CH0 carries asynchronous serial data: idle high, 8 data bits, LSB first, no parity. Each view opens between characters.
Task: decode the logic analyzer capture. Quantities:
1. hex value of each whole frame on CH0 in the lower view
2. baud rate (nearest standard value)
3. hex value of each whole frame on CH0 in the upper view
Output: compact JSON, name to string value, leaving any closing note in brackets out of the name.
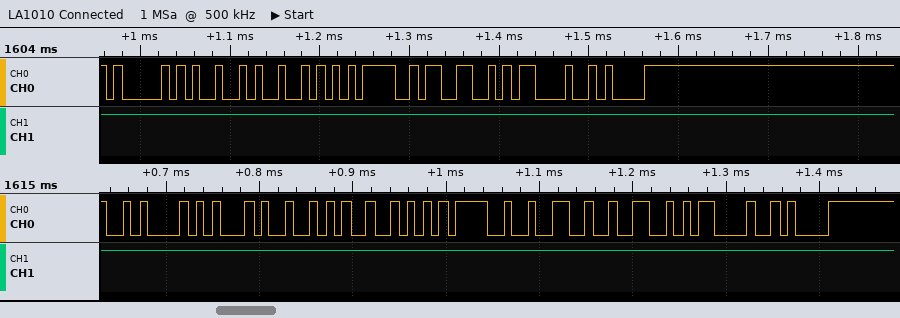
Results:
{"hex value of each whole frame on CH0 in the lower view": "0A, 45, 52, 52, 3D, 32, 32, 0D, 0A", "baud rate": "115200 baud", "hex value of each whole frame on CH0 in the upper view": "41, 49, 52, 3D, 33, 0D, 0A"}
